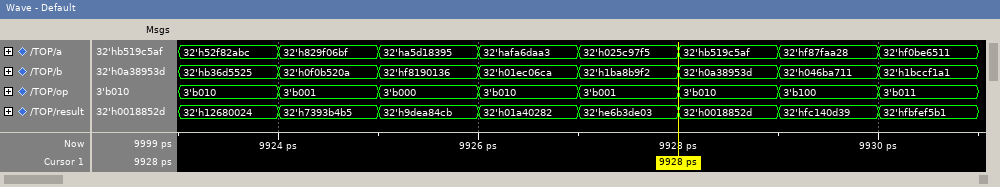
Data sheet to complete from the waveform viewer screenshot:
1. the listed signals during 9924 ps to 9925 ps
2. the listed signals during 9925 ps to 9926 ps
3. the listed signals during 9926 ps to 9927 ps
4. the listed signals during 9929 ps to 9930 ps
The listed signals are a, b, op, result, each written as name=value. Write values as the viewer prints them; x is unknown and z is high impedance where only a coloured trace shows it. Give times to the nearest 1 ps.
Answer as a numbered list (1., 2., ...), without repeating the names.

1. a=32'h829f06bf, b=32'h0f0b520a, op=3'b001, result=32'h7393b4b5
2. a=32'ha5d18395, b=32'hf8190136, op=3'b000, result=32'h9dea84cb
3. a=32'hafa6daa3, b=32'h01ec06ca, op=3'b010, result=32'h01a40282
4. a=32'hf87faa28, b=32'h046ba711, op=3'b100, result=32'hfc140d39
